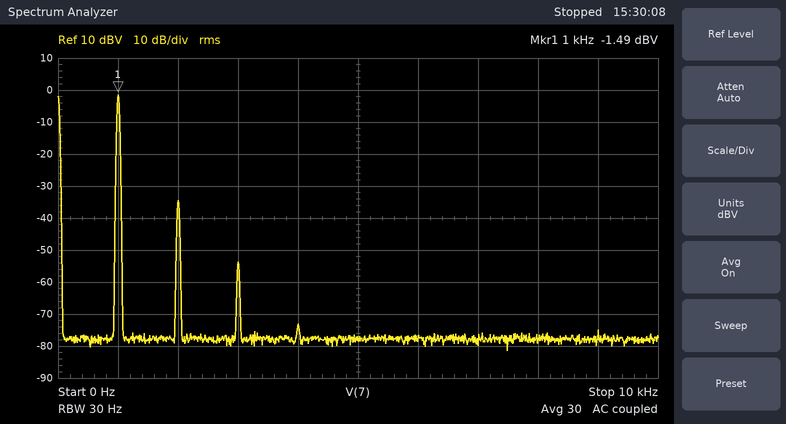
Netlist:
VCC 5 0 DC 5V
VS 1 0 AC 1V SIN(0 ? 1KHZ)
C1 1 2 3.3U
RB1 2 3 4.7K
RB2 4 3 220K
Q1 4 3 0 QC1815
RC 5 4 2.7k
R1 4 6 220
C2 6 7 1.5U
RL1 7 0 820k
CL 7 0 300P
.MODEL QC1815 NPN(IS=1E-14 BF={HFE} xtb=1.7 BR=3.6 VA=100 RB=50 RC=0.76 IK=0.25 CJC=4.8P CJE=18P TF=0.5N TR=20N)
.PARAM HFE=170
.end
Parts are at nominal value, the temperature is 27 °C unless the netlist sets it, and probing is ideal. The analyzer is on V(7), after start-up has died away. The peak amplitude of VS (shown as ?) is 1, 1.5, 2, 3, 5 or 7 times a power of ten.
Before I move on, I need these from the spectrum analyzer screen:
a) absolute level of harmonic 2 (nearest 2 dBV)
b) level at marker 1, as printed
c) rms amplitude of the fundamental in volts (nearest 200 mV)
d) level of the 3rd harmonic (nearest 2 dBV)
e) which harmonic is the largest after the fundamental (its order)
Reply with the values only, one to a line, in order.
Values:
-34 dBV
-1.49 dBV
800 mV
-54 dBV
2
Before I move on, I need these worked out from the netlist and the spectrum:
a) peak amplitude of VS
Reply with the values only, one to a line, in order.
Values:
50 mV
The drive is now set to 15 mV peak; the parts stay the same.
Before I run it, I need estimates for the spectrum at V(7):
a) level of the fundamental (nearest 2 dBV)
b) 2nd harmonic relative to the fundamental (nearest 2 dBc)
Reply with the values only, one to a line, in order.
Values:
-12 dBV
-44 dBc
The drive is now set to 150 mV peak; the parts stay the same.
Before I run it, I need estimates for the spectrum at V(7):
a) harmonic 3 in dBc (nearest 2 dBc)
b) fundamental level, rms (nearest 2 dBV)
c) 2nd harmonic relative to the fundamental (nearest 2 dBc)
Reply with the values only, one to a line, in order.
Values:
-18 dBc
6 dBV
-42 dBc
